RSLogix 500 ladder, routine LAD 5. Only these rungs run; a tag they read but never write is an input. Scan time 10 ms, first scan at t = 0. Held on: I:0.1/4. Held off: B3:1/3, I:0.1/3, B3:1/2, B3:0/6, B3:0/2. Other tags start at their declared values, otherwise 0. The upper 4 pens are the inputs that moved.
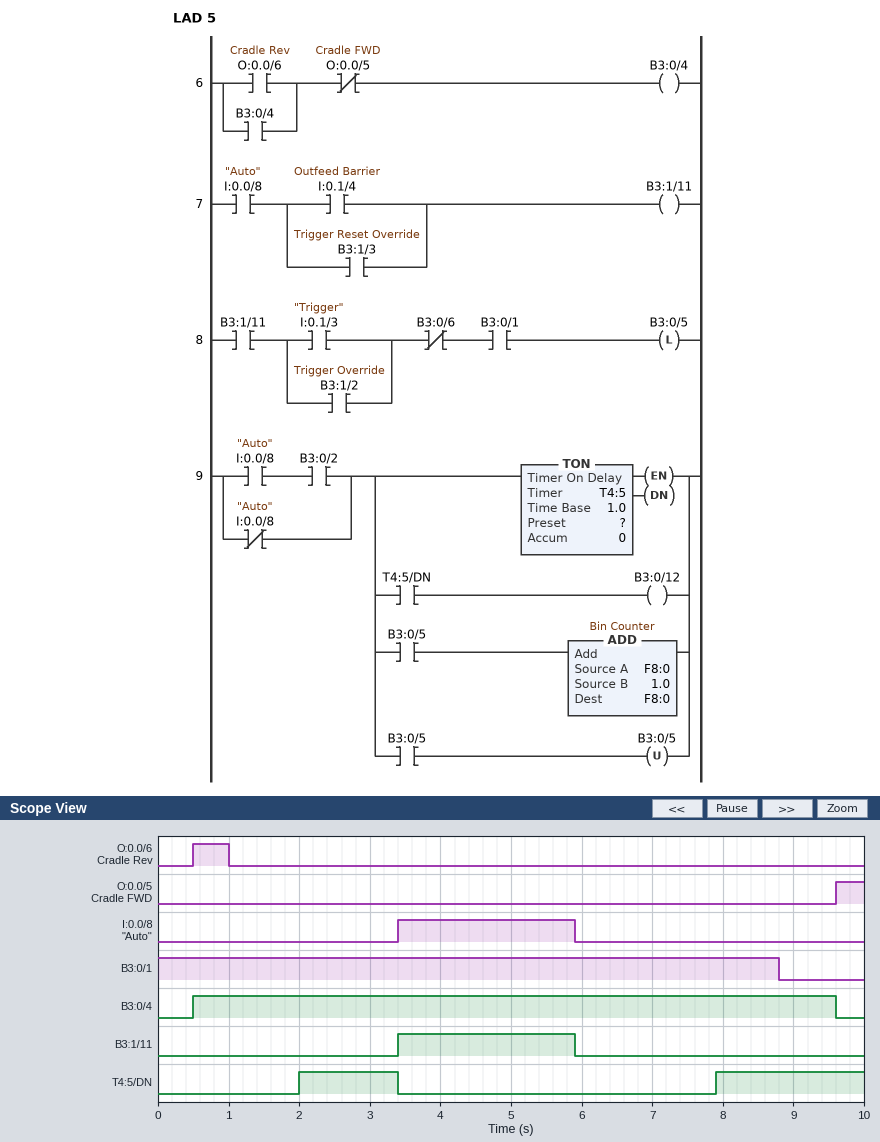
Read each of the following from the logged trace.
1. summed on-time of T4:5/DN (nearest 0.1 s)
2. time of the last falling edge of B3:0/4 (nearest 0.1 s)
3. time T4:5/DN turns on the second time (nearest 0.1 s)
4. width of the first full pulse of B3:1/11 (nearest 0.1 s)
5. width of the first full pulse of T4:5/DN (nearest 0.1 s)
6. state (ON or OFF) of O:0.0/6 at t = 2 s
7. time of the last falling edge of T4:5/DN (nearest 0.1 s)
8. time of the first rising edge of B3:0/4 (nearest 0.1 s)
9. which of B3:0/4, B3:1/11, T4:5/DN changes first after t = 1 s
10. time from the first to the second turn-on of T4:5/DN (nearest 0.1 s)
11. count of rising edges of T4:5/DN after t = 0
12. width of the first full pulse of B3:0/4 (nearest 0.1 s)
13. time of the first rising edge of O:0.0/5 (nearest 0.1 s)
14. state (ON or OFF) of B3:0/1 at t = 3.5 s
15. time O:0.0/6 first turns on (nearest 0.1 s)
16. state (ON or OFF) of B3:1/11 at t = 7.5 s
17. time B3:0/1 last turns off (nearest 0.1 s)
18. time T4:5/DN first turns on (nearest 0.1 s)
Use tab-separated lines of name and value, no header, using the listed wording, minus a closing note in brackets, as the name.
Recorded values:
summed on-time of T4:5/DN	3.5 s
time of the last falling edge of B3:0/4	9.6 s
time T4:5/DN turns on the second time	7.9 s
width of the first full pulse of B3:1/11	2.5 s
width of the first full pulse of T4:5/DN	1.4 s
state (ON or OFF) of O:0.0/6 at t = 2 s	OFF
time of the last falling edge of T4:5/DN	3.4 s
time of the first rising edge of B3:0/4	0.5 s
which of B3:0/4, B3:1/11, T4:5/DN changes first after t = 1 s	T4:5/DN
time from the first to the second turn-on of T4:5/DN	5.9 s
count of rising edges of T4:5/DN after t = 0	2
width of the first full pulse of B3:0/4	9.1 s
time of the first rising edge of O:0.0/5	9.6 s
state (ON or OFF) of B3:0/1 at t = 3.5 s	ON
time O:0.0/6 first turns on	0.5 s
state (ON or OFF) of B3:1/11 at t = 7.5 s	OFF
time B3:0/1 last turns off	8.8 s
time T4:5/DN first turns on	2.0 s
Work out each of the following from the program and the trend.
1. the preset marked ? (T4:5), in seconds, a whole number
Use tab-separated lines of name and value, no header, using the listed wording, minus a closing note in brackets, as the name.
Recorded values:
the preset marked ? (T4:5), in seconds, a whole number	2 s
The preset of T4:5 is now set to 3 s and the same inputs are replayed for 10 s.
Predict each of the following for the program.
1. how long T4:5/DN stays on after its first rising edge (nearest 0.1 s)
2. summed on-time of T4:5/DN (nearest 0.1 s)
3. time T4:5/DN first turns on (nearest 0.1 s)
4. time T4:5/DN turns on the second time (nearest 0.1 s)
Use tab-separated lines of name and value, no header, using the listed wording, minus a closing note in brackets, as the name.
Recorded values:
how long T4:5/DN stays on after its first rising edge	0.4 s
summed on-time of T4:5/DN	1.5 s
time T4:5/DN first turns on	3.0 s
time T4:5/DN turns on the second time	8.9 s
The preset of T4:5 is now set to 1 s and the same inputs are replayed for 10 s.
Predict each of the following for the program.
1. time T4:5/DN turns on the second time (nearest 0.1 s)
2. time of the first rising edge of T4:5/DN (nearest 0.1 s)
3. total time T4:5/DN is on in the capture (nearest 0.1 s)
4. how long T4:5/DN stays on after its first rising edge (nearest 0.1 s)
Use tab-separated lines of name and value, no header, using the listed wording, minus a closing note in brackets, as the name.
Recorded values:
time T4:5/DN turns on the second time	6.9 s
time of the first rising edge of T4:5/DN	1.0 s
total time T4:5/DN is on in the capture	5.5 s
how long T4:5/DN stays on after its first rising edge	2.4 s
